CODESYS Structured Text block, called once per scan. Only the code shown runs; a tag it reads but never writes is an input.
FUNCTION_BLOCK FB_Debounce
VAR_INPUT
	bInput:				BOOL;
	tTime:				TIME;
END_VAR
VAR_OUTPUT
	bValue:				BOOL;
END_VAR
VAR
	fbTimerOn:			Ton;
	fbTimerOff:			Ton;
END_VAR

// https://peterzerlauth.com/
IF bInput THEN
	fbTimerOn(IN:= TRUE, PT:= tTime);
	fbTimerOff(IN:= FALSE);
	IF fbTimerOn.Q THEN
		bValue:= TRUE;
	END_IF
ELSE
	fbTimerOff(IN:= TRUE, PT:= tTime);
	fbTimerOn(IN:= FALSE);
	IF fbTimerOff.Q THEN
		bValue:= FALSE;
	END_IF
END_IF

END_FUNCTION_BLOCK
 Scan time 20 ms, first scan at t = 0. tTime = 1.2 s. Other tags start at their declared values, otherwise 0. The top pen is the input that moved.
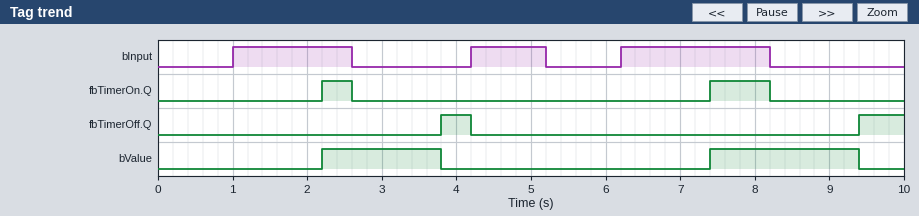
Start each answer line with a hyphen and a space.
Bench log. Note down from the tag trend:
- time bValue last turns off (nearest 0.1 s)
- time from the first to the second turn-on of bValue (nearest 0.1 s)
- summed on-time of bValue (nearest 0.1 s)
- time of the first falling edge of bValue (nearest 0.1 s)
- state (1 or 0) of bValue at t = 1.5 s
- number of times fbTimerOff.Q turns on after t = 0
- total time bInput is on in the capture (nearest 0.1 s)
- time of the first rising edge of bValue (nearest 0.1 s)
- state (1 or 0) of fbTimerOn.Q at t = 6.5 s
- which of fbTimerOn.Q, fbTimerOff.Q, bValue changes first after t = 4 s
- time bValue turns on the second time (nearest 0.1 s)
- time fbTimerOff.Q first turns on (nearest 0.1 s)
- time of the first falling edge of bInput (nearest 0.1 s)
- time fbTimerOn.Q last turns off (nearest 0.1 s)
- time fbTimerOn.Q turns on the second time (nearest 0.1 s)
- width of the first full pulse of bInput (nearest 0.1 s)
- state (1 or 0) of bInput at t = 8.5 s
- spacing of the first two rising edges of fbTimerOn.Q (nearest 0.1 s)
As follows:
- 9.4 s
- 5.2 s
- 3.6 s
- 3.8 s
- 0
- 2
- 4.6 s
- 2.2 s
- 0
- fbTimerOff.Q
- 7.4 s
- 3.8 s
- 2.6 s
- 8.2 s
- 7.4 s
- 1.6 s
- 0
- 5.2 s
